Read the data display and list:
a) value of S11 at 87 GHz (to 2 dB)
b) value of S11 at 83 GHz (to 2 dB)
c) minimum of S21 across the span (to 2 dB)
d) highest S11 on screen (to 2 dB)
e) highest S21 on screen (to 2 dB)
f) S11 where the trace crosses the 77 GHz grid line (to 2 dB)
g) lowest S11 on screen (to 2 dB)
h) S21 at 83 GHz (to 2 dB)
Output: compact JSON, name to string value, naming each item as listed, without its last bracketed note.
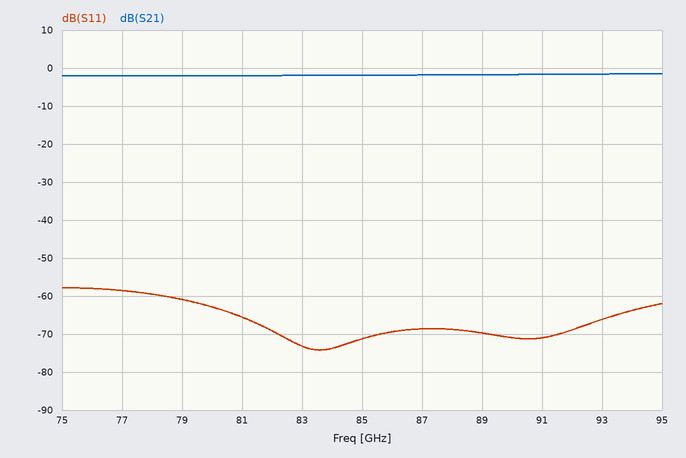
{"value of S11 at 87 GHz": "-68 dB", "value of S11 at 83 GHz": "-74 dB", "minimum of S21 across the span": "-2 dB", "highest S11 on screen": "-58 dB", "highest S21 on screen": "-2 dB", "S11 where the trace crosses the 77 GHz grid line": "-58 dB", "lowest S11 on screen": "-74 dB", "S21 at 83 GHz": "-2 dB"}
